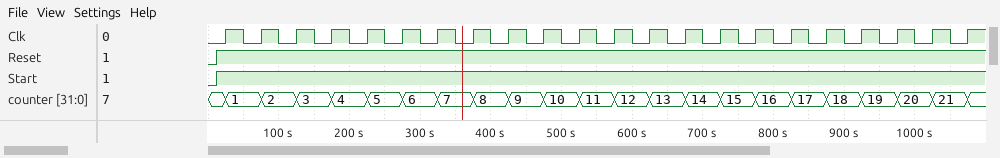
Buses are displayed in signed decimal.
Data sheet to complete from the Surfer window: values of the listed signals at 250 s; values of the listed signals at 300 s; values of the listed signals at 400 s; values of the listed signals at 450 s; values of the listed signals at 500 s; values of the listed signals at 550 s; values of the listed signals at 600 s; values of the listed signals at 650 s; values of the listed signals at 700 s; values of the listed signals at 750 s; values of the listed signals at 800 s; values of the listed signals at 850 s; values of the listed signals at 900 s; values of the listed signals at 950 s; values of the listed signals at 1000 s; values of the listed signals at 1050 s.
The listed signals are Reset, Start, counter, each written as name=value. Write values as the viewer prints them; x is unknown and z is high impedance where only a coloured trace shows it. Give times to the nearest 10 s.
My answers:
Reset=1, Start=1, counter=5
Reset=1, Start=1, counter=6
Reset=1, Start=1, counter=8
Reset=1, Start=1, counter=9
Reset=1, Start=1, counter=10
Reset=1, Start=1, counter=11
Reset=1, Start=1, counter=12
Reset=1, Start=1, counter=13
Reset=1, Start=1, counter=14
Reset=1, Start=1, counter=15
Reset=1, Start=1, counter=16
Reset=1, Start=1, counter=17
Reset=1, Start=1, counter=18
Reset=1, Start=1, counter=19
Reset=1, Start=1, counter=20
Reset=1, Start=1, counter=21
